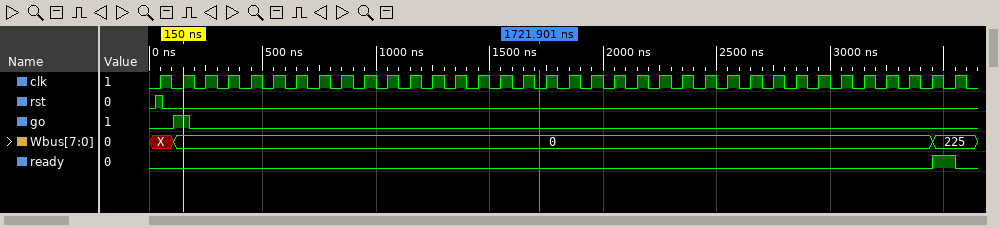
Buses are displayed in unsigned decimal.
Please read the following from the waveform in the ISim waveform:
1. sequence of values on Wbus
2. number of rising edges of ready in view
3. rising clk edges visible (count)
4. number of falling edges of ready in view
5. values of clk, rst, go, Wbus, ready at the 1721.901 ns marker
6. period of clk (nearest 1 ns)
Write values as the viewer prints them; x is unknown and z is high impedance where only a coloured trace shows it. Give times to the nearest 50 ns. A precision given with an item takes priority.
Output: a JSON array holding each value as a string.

["X, 0, 225", "1", "36", "1", "clk=0, rst=0, go=0, Wbus=0, ready=0", "100 ns"]
